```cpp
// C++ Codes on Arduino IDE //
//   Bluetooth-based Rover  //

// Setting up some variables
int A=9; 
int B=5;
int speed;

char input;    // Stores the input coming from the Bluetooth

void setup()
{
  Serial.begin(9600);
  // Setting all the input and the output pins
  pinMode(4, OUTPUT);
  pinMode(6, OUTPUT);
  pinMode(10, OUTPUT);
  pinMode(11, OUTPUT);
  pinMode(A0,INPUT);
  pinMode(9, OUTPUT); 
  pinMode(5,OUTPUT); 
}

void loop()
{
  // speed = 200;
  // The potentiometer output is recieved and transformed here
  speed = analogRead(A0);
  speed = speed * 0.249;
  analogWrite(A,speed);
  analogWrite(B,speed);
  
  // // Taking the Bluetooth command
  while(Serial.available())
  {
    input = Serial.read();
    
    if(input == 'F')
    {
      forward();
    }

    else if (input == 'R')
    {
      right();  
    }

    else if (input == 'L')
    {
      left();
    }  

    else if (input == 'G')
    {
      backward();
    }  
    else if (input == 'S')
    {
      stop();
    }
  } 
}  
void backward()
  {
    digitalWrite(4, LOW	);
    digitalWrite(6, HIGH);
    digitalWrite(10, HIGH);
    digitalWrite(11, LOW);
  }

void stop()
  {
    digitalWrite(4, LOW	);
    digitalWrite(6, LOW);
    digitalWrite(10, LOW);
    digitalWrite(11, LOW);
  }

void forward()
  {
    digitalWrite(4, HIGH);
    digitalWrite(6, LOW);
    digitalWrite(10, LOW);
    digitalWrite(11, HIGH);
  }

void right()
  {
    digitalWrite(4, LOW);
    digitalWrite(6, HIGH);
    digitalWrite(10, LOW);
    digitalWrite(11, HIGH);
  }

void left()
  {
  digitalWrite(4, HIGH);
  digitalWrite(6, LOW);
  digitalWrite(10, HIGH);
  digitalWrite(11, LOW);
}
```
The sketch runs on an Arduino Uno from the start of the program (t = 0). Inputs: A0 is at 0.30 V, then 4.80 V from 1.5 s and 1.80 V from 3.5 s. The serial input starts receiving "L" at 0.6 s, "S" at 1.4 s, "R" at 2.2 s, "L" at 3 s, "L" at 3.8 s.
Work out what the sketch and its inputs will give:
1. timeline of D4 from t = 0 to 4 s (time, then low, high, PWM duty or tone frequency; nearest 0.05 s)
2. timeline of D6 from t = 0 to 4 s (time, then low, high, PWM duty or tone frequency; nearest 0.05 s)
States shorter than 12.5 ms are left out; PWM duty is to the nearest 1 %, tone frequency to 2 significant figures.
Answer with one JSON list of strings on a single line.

["0 s low; 0.6 s high; 1.4 s low; 3 s high", "0 s low; 2.2 s high; 3 s low"]
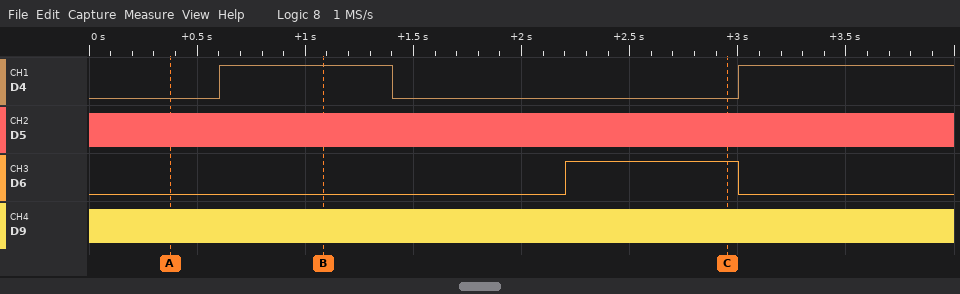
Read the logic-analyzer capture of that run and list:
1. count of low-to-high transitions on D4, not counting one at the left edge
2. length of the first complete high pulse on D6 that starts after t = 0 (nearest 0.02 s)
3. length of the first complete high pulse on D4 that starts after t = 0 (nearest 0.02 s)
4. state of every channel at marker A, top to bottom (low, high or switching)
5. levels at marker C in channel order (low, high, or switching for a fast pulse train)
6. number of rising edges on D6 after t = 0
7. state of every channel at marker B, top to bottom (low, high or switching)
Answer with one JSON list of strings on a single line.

["2", "0.80 s", "0.80 s", "D4 low, D5 switching, D6 low, D9 switching", "D4 low, D5 switching, D6 high, D9 switching", "1", "D4 high, D5 switching, D6 low, D9 switching"]
